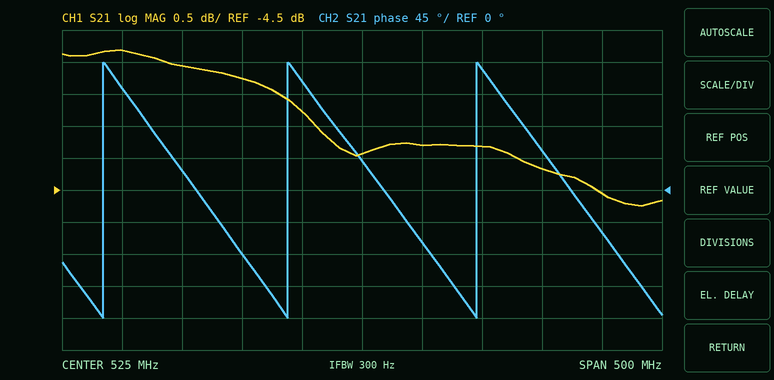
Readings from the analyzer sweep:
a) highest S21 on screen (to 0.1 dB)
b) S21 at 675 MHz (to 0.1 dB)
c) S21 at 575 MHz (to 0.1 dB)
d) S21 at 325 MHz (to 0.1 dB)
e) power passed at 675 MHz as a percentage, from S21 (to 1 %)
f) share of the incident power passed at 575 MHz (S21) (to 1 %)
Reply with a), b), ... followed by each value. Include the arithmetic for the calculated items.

a) -2.3 dB
b) -4.2 dB
c) -3.8 dB
d) -2.3 dB
e) 10^(-4.2/10) ≈ 38 %
f) 10^(-3.8/10) ≈ 42 %
